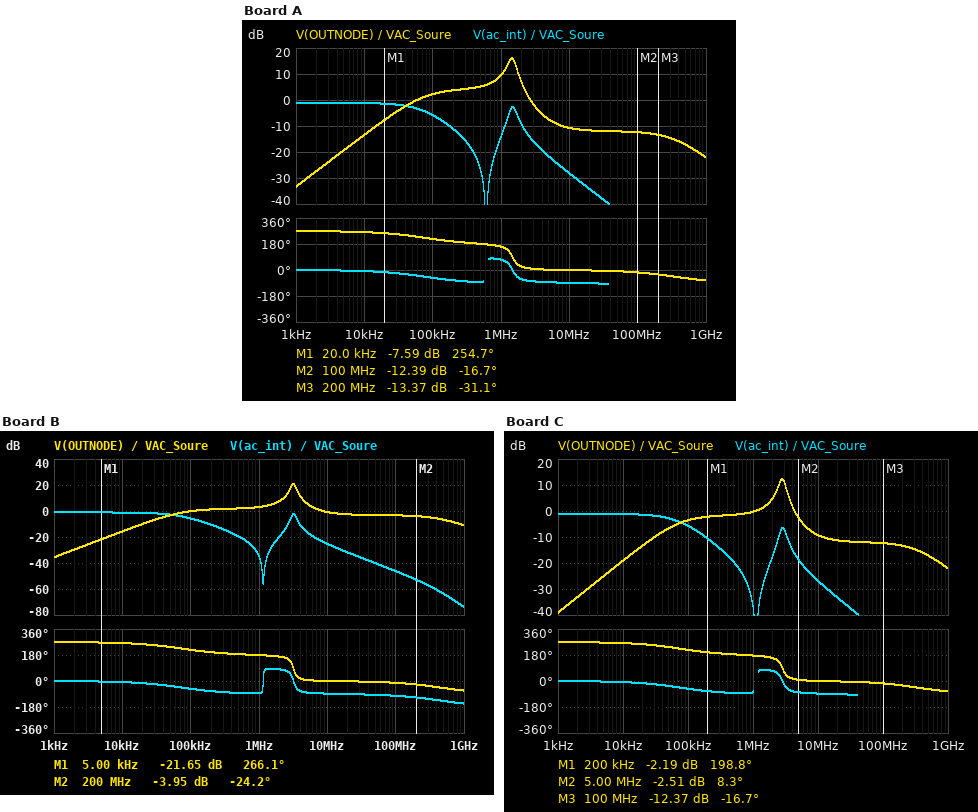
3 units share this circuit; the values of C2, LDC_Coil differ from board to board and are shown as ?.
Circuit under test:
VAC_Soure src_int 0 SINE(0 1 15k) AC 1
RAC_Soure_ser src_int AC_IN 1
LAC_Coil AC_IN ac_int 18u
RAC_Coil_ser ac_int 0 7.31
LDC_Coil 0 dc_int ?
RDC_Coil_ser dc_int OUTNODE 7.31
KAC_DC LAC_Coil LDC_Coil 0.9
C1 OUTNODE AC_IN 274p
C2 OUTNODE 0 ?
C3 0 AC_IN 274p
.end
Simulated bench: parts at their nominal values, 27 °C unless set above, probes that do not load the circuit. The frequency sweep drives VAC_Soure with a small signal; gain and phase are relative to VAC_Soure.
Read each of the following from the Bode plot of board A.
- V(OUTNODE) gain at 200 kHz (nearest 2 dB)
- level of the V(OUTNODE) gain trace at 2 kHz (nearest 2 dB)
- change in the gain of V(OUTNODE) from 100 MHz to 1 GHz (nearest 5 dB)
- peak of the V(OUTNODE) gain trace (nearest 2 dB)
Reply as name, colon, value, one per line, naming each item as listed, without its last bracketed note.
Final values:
V(OUTNODE) gain at 200 kHz: 4 dB
level of the V(OUTNODE) gain trace at 2 kHz: -28 dB
change in the gain of V(OUTNODE) from 100 MHz to 1 GHz: -10 dB
peak of the V(OUTNODE) gain trace: 16 dB
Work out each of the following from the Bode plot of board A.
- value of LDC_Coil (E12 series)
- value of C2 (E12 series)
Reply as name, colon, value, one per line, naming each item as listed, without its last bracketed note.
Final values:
value of LDC_Coil: 56 µH
value of C2: 820 pF
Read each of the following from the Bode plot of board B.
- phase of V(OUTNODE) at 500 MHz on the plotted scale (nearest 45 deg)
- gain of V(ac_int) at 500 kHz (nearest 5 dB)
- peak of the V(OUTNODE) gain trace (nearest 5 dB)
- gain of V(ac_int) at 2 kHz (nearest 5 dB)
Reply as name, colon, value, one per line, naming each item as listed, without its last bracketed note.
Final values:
phase of V(OUTNODE) at 500 MHz on the plotted scale: -45 deg
gain of V(ac_int) at 500 kHz: -20 dB
peak of the V(OUTNODE) gain trace: 20 dB
gain of V(ac_int) at 2 kHz: 0 dB
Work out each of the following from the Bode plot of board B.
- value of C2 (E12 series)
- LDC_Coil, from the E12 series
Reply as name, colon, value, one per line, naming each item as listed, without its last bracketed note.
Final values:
value of C2: 120 pF
LDC_Coil, from the E12 series: 33 µH
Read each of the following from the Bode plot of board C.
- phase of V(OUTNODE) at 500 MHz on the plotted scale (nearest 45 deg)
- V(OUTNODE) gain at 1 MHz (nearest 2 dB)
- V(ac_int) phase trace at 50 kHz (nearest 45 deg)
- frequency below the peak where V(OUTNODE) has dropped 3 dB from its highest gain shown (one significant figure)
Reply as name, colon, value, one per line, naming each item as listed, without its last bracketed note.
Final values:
phase of V(OUTNODE) at 500 MHz on the plotted scale: -45 deg
V(OUTNODE) gain at 1 MHz: 0 dB
V(ac_int) phase trace at 50 kHz: -45 deg
frequency below the peak where V(OUTNODE) has dropped 3 dB from its highest gain shown: 2 MHz
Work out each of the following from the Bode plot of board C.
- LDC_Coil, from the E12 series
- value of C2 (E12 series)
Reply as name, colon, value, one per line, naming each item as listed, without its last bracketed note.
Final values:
LDC_Coil, from the E12 series: 15 µH
value of C2: 820 pF
